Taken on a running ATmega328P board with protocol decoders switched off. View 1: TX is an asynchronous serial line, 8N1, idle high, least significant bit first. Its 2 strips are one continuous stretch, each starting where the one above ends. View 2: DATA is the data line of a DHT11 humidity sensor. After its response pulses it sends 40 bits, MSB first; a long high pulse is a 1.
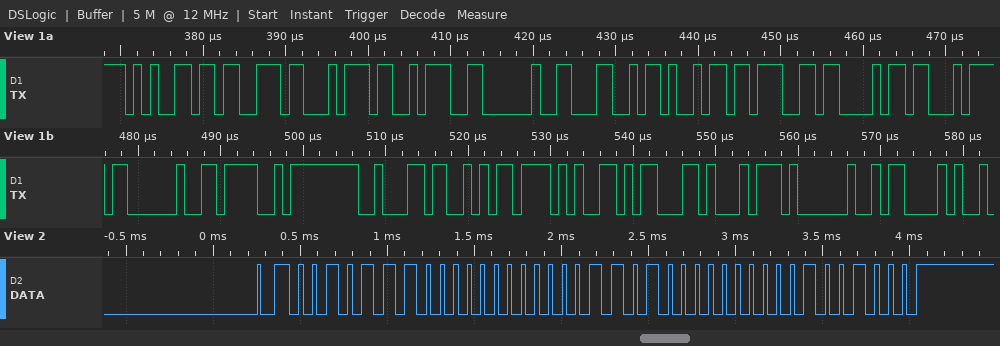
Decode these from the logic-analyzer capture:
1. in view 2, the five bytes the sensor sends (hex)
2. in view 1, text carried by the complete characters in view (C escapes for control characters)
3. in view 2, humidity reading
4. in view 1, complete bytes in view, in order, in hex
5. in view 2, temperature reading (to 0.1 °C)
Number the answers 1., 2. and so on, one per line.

1. 2E 00 1A 00 48
2. "est: Light Object C"
3. 46 %
4. 0x65 0x73 0x74 0x3A 0x20 0x4C 0x69 0x67 0x68 0x74 0x20 0x4F 0x62 0x6A 0x65 0x63 0x74 0x20 0x43
5. 26.0 °C
